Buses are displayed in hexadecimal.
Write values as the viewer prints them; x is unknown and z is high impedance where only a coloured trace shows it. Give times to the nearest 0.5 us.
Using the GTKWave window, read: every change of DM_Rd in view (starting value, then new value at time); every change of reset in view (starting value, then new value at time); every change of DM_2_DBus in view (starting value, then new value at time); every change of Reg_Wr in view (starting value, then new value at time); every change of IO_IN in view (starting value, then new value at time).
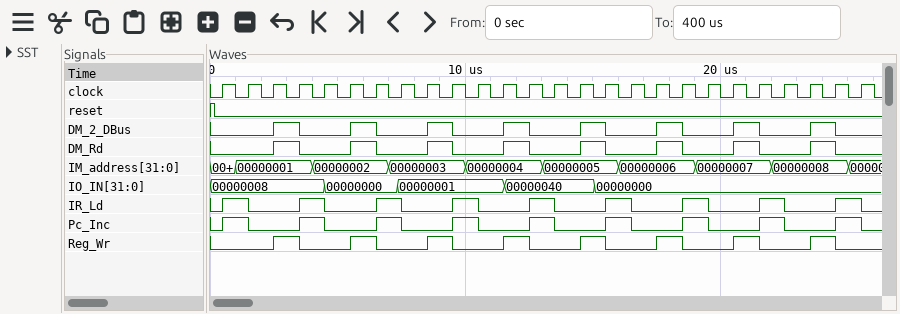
0, 1 at 2.5 us, 0 at 3.5 us, 1 at 5.5 us, 0 at 6.5 us, 1 at 8.5 us, 0 at 9.5 us, 1 at 11.5 us, 0 at 12.5 us, 1 at 14.5 us, 0 at 15.5 us, 1 at 17.5 us, 0 at 18.5 us, 1 at 20.5 us, 0 at 21.5 us, 1 at 23.5 us, 0 at 24.5 us
1, 0 at 0 us
0, 1 at 2.5 us, 0 at 3.5 us, 1 at 5.5 us, 0 at 6.5 us, 1 at 8.5 us, 0 at 9.5 us, 1 at 11.5 us, 0 at 12.5 us, 1 at 14.5 us, 0 at 15.5 us, 1 at 17.5 us, 0 at 18.5 us, 1 at 20.5 us, 0 at 21.5 us, 1 at 23.5 us, 0 at 24.5 us
0, 1 at 2.5 us, 0 at 3.5 us, 1 at 5.5 us, 0 at 6.5 us, 1 at 8.5 us, 0 at 9.5 us, 1 at 11.5 us, 0 at 12.5 us, 1 at 14.5 us, 0 at 15.5 us, 1 at 17.5 us, 0 at 18.5 us, 1 at 20.5 us, 0 at 21.5 us, 1 at 23.5 us, 0 at 24.5 us
00000008, 00000000 at 4.5 us, 00000001 at 7.5 us, 00000040 at 11.5 us, 00000000 at 15 us
